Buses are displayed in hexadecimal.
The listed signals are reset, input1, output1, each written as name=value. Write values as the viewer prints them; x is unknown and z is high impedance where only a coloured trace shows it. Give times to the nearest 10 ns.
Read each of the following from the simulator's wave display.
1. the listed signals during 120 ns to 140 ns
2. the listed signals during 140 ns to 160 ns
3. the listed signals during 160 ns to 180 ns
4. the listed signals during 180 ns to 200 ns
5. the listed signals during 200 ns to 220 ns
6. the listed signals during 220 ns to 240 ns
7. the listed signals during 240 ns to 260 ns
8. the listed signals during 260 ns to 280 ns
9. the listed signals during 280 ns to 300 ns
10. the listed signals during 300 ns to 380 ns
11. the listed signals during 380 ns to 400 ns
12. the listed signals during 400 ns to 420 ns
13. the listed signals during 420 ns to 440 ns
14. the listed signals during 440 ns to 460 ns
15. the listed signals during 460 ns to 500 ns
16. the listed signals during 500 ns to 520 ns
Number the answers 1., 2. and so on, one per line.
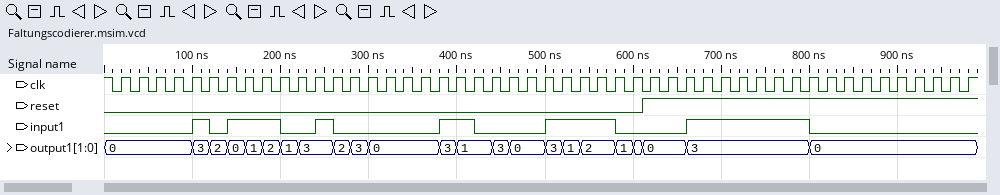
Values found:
1. reset=0, input1=0, output1=2
2. reset=0, input1=1, output1=0
3. reset=0, input1=1, output1=1
4. reset=0, input1=1, output1=2
5. reset=0, input1=0, output1=1
6. reset=0, input1=0, output1=3
7. reset=0, input1=1, output1=3
8. reset=0, input1=0, output1=2
9. reset=0, input1=0, output1=3
10. reset=0, input1=0, output1=0
11. reset=0, input1=1, output1=3
12. reset=0, input1=1, output1=1
13. reset=0, input1=0, output1=1
14. reset=0, input1=0, output1=3
15. reset=0, input1=0, output1=0
16. reset=0, input1=1, output1=3
